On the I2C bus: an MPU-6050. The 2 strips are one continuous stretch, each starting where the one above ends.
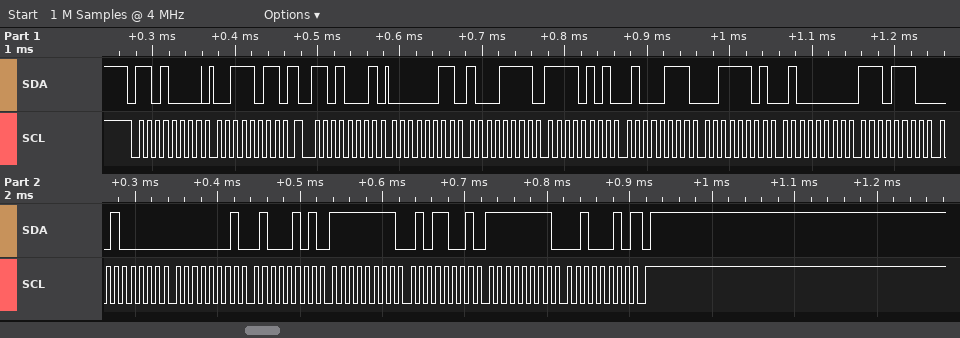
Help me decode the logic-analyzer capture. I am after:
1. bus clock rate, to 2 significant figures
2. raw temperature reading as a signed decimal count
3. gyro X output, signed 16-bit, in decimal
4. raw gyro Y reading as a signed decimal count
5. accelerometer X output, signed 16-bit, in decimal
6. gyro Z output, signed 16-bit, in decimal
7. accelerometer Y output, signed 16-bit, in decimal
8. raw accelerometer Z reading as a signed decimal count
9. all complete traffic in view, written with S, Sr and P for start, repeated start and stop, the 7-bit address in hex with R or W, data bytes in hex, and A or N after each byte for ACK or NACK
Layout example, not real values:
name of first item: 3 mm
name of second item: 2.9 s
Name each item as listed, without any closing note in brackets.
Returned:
bus clock rate, to 2 significant figures: 100 kHz
raw temperature reading as a signed decimal count: -4576
gyro X output, signed 16-bit, in decimal: 325
raw gyro Y reading as a signed decimal count: -167
accelerometer X output, signed 16-bit, in decimal: 911
gyro Z output, signed 16-bit, in decimal: -222
accelerometer Y output, signed 16-bit, in decimal: -2745
raw accelerometer Z reading as a signed decimal count: 15680
all complete traffic in view, written with S, Sr and P for start, repeated start and stop, the 7-bit address in hex with R or W, data bytes in hex, and A or N after each byte for ACK or NACK: S 68W A 3B A Sr 68R A 03 A 8F A F5 A 47 A 3D A 40 A EE A 20 A 01 A 45 A FF A 59 A FF A 22 N P
